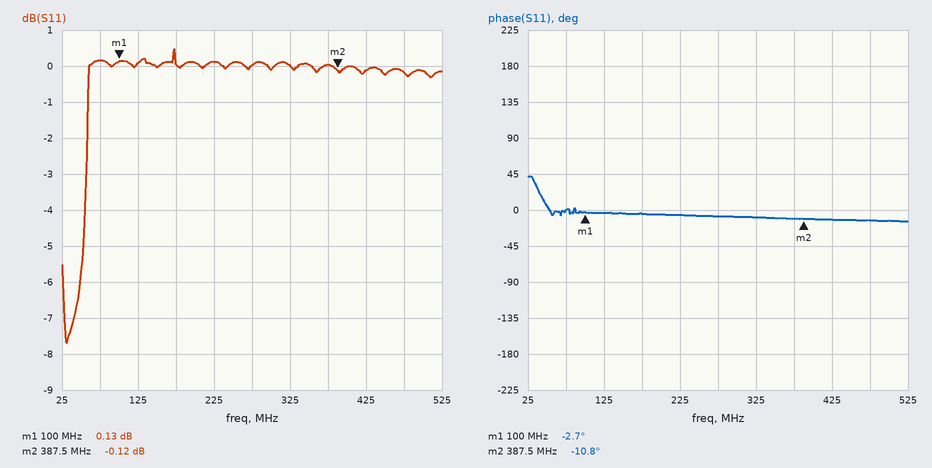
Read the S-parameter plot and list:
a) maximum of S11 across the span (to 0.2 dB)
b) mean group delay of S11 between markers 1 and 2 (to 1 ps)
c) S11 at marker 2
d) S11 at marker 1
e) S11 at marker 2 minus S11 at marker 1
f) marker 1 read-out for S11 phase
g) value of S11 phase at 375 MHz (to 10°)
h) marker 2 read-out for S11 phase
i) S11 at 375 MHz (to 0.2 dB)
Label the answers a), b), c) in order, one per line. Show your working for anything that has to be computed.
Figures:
a) 0.4 dB
b) −(-10.8° − (-2.7°))/(360° × 287.5 MHz) ≈ 78 ps
c) -0.12 dB
d) 0.13 dB
e) -0.12 − (0.13) = -0.25 dB
f) -2.7°
g) -10°
h) -10.8°
i) 0.0 dB
